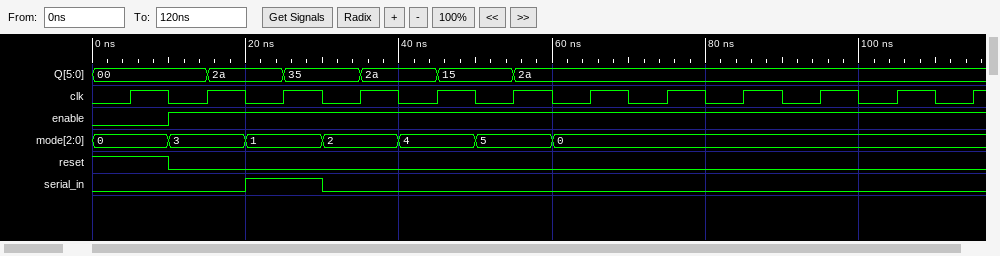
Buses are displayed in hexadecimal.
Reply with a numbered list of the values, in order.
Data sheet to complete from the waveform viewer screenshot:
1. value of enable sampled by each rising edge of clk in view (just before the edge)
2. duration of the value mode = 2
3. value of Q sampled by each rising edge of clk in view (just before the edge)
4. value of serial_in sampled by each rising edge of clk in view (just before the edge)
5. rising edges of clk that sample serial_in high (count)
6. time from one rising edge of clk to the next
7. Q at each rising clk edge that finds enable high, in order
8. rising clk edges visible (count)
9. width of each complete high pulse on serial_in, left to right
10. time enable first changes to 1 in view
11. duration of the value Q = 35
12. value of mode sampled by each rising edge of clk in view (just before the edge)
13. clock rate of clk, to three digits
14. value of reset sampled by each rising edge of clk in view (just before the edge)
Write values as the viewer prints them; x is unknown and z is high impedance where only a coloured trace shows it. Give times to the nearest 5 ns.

1. 0 1 1 1 1 1 1 1 1 1 1 1
2. 10 ns
3. 00, 00, 2a, 35, 2a, 15, 2a, 2a, 2a, 2a, 2a, 2a
4. 0 0 1 0 0 0 0 0 0 0 0 0
5. 1
6. 10 ns
7. 00, 2a, 35, 2a, 15, 2a, 2a, 2a, 2a, 2a, 2a
8. 12
9. 10 ns
10. 10 ns
11. 10 ns
12. 0, 3, 1, 2, 4, 5, 0, 0, 0, 0, 0, 0
13. 100 MHz
14. 1 0 0 0 0 0 0 0 0 0 0 0
